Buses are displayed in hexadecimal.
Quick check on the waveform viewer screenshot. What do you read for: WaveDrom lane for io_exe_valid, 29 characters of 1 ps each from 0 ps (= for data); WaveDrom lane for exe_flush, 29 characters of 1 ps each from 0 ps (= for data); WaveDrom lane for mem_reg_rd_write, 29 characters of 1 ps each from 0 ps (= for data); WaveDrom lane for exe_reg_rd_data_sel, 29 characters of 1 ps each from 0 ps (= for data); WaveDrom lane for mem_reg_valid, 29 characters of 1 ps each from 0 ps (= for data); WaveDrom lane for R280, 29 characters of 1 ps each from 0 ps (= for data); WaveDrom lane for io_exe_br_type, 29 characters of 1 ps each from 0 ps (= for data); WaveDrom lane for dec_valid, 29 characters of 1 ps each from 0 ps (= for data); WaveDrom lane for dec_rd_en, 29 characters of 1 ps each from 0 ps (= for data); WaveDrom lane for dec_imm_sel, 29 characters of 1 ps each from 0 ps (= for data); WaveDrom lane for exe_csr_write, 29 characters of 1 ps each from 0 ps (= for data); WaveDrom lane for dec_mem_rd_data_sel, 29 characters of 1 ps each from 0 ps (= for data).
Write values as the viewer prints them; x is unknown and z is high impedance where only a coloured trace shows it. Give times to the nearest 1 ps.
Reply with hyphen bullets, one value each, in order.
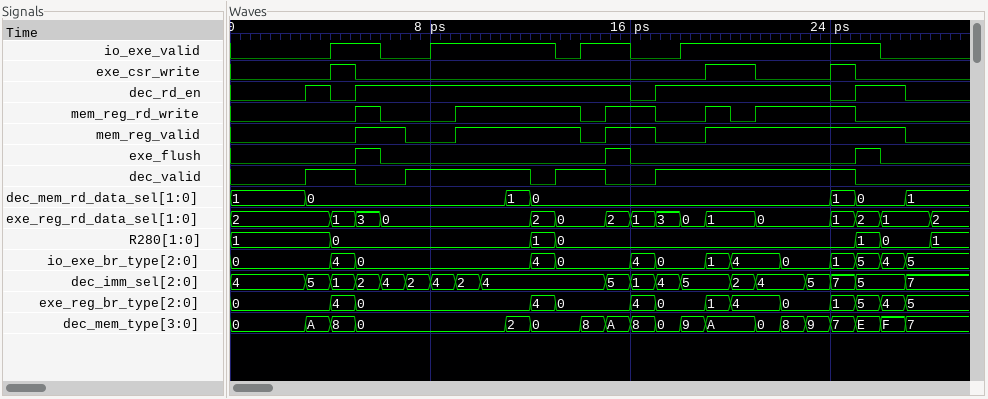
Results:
- {name: 'io_exe_valid', wave: '0...1.0.1....01.0.1.......0..'}
- {name: 'exe_flush', wave: '0....10........10........10..'}
- {name: 'mem_reg_rd_write', wave: '0....10..1....01.0.101...0...'}
- {name: 'exe_reg_rd_data_sel', wave: '=...===.....==.=====.=..===.=', data: '2 1 3 0 2 0 2 1 3 0 1 0 1 2 1 2'}
- {name: 'mem_reg_valid', wave: '0....1.0.1....01.0.1.......0.'}
- {name: 'R280', wave: '=...=.......==...........==.=', data: '1 0 1 0 1 0 1'}
- {name: 'io_exe_br_type', wave: '=...==......==..==.==.=.====.', data: '0 4 0 4 0 4 0 1 4 0 1 5 4 5'}
- {name: 'dec_valid', wave: '0..1.0.1....01.0.1.......0...'}
- {name: 'dec_rd_en', wave: '0..101..........01......01.0.'}
- {name: 'dec_imm_sel', wave: '=..========....====.==.===.=.', data: '4 5 1 2 4 2 4 2 4 5 1 4 5 2 4 5 7 5 7'}
- {name: 'exe_csr_write', wave: '0...10.............1.0..10...'}
- {name: 'dec_mem_rd_data_sel', wave: '=..=.......==...........==.=.', data: '1 0 1 0 1 0 1'}
